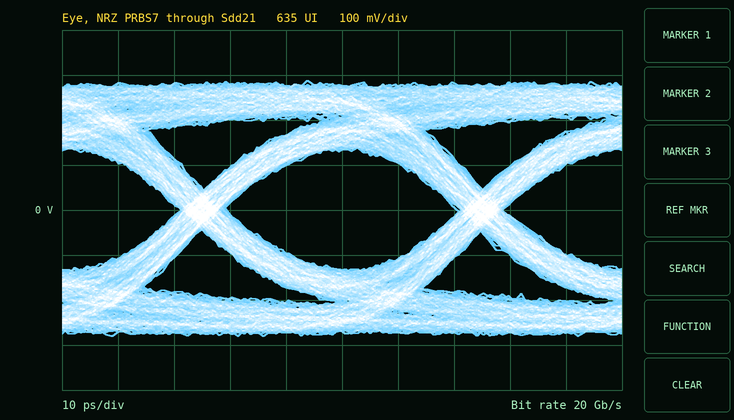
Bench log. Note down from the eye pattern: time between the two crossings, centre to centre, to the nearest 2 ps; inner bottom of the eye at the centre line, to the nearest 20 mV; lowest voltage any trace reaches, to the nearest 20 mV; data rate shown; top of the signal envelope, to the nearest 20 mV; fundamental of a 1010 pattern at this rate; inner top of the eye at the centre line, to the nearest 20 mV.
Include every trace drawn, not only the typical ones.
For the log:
50 ps
-140 mV
-280 mV
20 Gb/s
280 mV
10 GHz
140 mV
